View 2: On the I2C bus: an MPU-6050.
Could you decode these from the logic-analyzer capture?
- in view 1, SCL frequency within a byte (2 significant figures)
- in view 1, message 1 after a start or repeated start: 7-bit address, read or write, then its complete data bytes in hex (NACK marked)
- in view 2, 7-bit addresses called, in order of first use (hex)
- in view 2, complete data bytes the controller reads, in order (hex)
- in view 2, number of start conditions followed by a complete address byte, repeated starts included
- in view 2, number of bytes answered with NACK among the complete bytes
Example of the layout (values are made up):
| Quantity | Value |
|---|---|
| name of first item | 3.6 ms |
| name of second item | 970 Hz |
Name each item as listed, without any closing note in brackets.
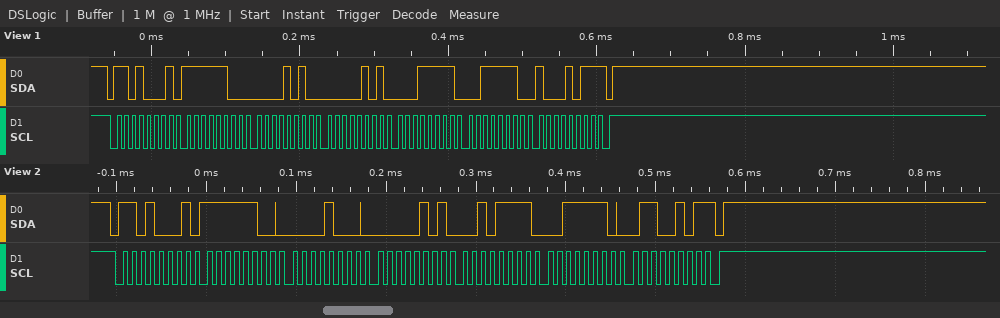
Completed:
| Quantity | Value |
|---|---|
| in view 1, SCL frequency within a byte | 100 kHz |
| in view 1, message 1 after a start or repeated start: 7-bit address, read or write, then its complete data bytes in hex | 0x68 read: FC 0A 05 1F 3E 8B NACK |
| in view 2, 7-bit addresses called, in order of first use | 0x68 |
| in view 2, complete data bytes the controller reads, in order | FC 08 05 2F 3E 65 |
| in view 2, number of start conditions followed by a complete address byte, repeated starts included | 1 |
| in view 2, number of bytes answered with NACK among the complete bytes | 1 |
